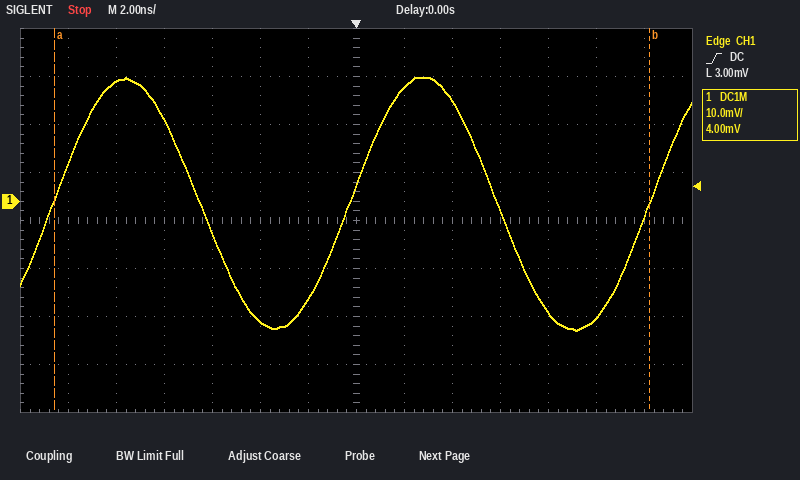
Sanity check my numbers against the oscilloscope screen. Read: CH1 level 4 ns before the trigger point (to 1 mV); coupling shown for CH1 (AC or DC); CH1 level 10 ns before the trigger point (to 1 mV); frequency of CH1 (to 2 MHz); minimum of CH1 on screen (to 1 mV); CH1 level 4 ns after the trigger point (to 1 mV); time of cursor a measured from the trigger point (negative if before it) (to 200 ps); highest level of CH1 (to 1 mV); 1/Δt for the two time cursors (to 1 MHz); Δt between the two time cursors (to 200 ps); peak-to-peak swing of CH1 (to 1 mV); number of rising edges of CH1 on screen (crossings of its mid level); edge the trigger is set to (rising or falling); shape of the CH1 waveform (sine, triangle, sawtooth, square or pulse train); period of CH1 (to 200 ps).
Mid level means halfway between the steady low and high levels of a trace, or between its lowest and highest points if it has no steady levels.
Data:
-25 mV
DC
25 mV
80 MHz
-27 mV
21 mV
-12.6 ns
26 mV
40 MHz
24.8 ns
53 mV
3
rising
sine
12.4 ns
